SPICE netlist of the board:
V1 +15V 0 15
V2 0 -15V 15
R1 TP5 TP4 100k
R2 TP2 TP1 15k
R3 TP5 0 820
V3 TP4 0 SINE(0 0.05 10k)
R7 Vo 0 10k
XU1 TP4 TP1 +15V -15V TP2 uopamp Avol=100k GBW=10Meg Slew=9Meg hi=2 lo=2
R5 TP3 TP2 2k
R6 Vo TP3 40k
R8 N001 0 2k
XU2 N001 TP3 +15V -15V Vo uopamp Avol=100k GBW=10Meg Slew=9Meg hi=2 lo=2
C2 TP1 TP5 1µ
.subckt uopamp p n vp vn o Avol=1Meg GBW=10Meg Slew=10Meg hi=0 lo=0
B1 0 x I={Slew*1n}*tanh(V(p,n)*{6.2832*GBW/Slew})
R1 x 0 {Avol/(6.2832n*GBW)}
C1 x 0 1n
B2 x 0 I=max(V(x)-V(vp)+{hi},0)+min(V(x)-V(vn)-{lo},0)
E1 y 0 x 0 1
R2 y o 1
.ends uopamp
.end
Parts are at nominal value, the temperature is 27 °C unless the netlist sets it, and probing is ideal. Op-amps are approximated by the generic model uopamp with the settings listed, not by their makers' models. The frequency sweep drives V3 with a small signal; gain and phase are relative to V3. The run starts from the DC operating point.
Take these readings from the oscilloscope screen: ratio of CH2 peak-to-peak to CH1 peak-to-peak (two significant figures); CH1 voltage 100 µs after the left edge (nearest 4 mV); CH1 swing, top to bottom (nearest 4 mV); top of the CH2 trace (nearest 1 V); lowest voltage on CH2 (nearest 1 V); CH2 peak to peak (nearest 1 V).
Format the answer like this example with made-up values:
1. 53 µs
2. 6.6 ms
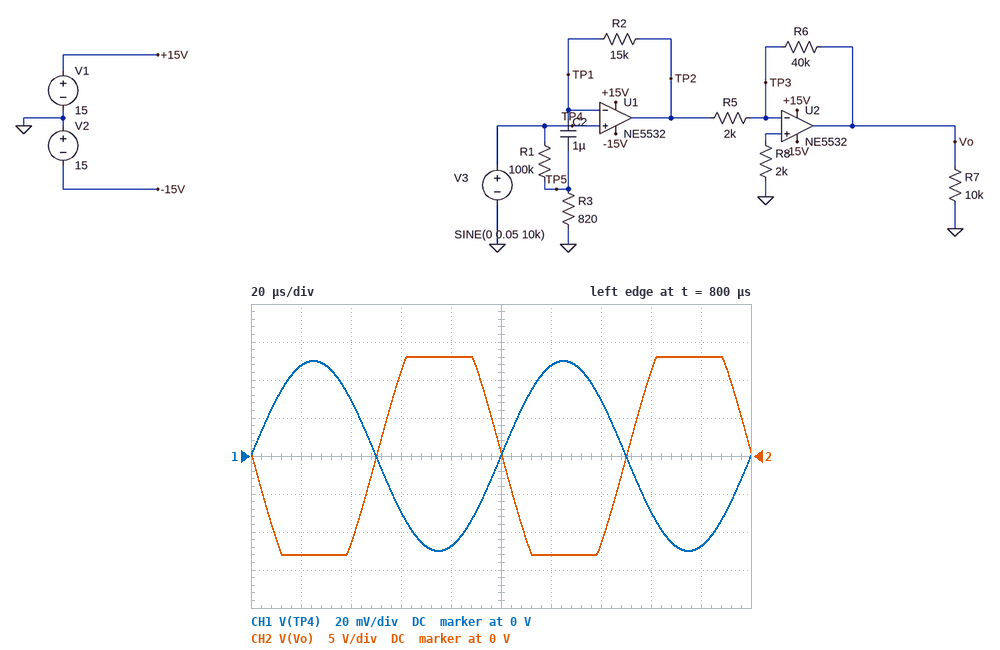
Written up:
1. 260
2. 0 V
3. 100 mV
4. 13 V
5. -13 V
6. 26 V
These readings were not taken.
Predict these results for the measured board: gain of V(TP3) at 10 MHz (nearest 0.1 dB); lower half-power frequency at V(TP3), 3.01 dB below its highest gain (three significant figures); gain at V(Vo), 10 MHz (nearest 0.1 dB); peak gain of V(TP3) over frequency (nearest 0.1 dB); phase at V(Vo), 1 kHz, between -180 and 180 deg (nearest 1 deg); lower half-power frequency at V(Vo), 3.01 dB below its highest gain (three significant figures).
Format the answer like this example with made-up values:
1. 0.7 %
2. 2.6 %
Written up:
1. -0.5 dB
2. 205 kHz
3. -0.5 dB
4. 19.6 dB
5. -170 deg
6. 195 Hz
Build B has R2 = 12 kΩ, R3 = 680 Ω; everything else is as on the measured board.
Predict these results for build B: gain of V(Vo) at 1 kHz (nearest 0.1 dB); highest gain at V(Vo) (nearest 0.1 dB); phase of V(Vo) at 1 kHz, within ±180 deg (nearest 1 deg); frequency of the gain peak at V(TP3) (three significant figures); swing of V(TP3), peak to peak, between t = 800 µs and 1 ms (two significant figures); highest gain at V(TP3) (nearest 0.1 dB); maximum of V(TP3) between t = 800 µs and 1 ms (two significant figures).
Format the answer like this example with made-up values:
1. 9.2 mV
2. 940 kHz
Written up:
1. 51.2 dB
2. 51.4 dB
3. -168 deg
4. 504 kHz
5. 540 mV
6. 19.4 dB
7. 260 mV
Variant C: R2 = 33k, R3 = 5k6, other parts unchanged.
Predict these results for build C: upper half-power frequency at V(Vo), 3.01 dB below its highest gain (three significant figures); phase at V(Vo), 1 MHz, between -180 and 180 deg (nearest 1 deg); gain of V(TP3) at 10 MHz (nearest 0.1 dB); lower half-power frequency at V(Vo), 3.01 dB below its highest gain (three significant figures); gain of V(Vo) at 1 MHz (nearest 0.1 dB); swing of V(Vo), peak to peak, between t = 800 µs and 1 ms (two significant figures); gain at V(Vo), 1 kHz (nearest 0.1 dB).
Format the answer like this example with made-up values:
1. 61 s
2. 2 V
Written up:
1. 432 kHz
2. 80 deg
3. -0.9 dB
4. 29.4 Hz
5. 33.6 dB
6. 14 V
7. 42.8 dB
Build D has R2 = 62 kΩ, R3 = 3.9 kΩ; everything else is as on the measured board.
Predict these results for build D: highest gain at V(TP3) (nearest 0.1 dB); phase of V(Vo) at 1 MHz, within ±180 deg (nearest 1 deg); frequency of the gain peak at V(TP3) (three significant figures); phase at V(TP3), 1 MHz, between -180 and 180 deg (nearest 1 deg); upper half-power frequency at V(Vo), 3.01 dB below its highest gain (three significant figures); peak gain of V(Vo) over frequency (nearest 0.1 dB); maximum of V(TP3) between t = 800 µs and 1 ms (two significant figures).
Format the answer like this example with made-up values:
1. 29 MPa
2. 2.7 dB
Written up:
1. 18.9 dB
2. 55 deg
3. 521 kHz
4. -35 deg
5. 334 kHz
6. 50.6 dB
7. 180 mV
